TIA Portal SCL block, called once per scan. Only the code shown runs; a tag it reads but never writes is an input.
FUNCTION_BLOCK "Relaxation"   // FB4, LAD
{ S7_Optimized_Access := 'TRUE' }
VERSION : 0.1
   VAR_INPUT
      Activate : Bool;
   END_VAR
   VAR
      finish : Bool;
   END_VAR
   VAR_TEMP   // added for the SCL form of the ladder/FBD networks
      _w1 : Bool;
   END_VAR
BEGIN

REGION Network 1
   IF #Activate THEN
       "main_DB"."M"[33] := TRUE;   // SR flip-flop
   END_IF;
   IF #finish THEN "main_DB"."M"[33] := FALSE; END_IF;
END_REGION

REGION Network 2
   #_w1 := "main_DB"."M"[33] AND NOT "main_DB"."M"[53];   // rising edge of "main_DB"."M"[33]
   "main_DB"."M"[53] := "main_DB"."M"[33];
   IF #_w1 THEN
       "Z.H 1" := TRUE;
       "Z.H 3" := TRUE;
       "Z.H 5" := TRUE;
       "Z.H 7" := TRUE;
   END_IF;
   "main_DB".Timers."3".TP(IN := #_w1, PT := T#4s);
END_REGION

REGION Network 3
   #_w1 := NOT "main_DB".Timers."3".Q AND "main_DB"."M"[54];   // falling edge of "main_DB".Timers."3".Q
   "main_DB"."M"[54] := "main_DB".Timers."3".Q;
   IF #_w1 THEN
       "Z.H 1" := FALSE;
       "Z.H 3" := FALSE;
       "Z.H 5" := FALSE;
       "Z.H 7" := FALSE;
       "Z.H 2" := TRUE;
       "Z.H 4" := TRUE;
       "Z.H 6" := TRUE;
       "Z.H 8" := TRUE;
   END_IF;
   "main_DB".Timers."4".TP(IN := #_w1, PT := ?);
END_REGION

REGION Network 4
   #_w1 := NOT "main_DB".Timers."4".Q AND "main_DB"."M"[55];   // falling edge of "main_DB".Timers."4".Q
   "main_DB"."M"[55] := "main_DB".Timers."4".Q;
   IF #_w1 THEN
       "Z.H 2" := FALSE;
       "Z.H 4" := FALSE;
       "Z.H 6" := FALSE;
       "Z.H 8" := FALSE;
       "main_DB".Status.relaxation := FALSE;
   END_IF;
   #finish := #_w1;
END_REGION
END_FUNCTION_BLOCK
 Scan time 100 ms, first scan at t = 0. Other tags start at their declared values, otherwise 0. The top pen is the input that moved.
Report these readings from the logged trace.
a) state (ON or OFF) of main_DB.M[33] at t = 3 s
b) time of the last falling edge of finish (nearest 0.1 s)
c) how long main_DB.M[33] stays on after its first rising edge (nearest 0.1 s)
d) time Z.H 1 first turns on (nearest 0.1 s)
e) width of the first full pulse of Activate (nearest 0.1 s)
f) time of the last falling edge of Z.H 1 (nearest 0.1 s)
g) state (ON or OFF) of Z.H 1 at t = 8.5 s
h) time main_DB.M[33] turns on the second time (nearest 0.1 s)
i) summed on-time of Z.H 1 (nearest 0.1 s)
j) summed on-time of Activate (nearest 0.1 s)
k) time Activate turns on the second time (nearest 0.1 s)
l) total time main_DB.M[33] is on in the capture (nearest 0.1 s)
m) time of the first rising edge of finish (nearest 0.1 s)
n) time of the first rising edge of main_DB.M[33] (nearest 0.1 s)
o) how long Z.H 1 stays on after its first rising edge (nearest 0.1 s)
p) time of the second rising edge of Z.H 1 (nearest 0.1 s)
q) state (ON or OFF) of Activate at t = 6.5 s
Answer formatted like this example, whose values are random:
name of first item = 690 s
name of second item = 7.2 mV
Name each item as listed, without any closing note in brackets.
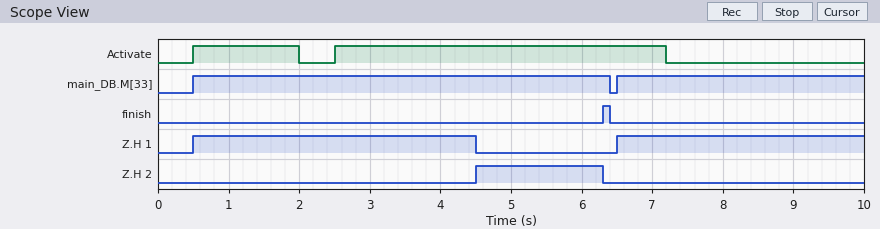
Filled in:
state (ON or OFF) of main_DB.M[33] at t = 3 s = ON
time of the last falling edge of finish = 6.4 s
how long main_DB.M[33] stays on after its first rising edge = 5.9 s
time Z.H 1 first turns on = 0.5 s
width of the first full pulse of Activate = 1.5 s
time of the last falling edge of Z.H 1 = 4.5 s
state (ON or OFF) of Z.H 1 at t = 8.5 s = ON
time main_DB.M[33] turns on the second time = 6.5 s
summed on-time of Z.H 1 = 7.5 s
summed on-time of Activate = 6.2 s
time Activate turns on the second time = 2.5 s
total time main_DB.M[33] is on in the capture = 9.4 s
time of the first rising edge of finish = 6.3 s
time of the first rising edge of main_DB.M[33] = 0.5 s
how long Z.H 1 stays on after its first rising edge = 4.0 s
time of the second rising edge of Z.H 1 = 6.5 s
state (ON or OFF) of Activate at t = 6.5 s = ON
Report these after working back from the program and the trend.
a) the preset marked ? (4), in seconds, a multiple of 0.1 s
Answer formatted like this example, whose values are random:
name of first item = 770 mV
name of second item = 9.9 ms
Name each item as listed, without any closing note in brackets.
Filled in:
the preset marked ? (4), in seconds, a multiple of 0.1 s = 1.8 s
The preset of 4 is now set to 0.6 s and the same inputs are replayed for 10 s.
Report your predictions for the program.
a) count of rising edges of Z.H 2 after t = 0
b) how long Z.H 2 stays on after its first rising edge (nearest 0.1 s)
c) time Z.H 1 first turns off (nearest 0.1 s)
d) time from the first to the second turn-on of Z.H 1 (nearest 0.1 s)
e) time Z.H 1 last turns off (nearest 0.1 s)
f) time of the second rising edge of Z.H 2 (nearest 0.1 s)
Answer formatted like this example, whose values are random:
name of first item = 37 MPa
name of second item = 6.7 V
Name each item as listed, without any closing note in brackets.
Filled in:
count of rising edges of Z.H 2 after t = 0 = 2
how long Z.H 2 stays on after its first rising edge = 0.6 s
time Z.H 1 first turns off = 4.5 s
time from the first to the second turn-on of Z.H 1 = 4.8 s
time Z.H 1 last turns off = 9.3 s
time of the second rising edge of Z.H 2 = 9.3 s
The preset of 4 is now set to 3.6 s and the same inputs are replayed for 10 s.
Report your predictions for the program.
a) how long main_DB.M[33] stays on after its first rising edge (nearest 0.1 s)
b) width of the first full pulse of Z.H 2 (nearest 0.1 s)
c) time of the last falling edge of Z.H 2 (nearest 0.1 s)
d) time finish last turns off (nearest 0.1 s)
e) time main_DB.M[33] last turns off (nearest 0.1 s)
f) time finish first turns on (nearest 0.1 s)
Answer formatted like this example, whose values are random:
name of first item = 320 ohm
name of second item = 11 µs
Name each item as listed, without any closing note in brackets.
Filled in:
how long main_DB.M[33] stays on after its first rising edge = 7.7 s
width of the first full pulse of Z.H 2 = 3.6 s
time of the last falling edge of Z.H 2 = 8.1 s
time finish last turns off = 8.2 s
time main_DB.M[33] last turns off = 8.2 s
time finish first turns on = 8.1 s
